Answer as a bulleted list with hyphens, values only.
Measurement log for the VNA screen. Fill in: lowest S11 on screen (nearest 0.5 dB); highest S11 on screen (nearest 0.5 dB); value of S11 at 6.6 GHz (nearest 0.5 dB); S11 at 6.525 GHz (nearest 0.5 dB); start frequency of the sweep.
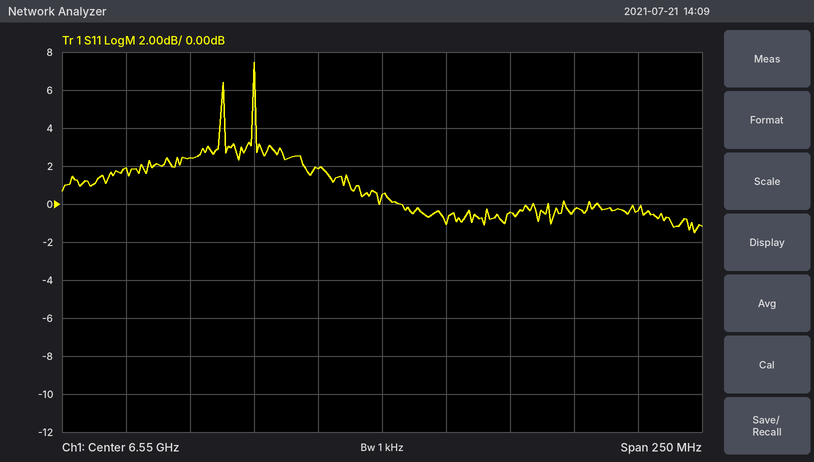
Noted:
- -1.5 dB
- 7.5 dB
- -0.5 dB
- 2.0 dB
- 6.425 GHz
